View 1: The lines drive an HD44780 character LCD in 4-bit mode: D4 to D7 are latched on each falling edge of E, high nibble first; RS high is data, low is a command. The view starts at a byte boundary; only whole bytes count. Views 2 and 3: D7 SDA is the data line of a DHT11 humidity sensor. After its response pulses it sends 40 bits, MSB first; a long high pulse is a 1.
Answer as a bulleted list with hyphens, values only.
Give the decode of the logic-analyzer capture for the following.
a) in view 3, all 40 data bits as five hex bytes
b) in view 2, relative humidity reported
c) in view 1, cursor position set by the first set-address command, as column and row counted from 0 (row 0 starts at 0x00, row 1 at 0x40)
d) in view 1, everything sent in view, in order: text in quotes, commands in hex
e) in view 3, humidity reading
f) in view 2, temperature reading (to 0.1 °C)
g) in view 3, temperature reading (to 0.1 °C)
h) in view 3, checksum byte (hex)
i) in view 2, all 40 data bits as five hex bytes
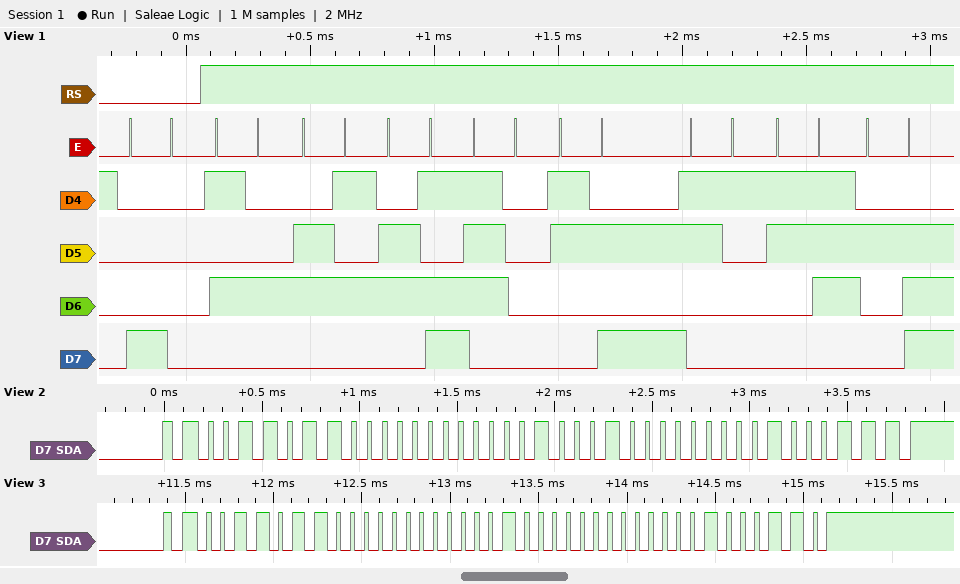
- 36 00 10 00 46
- 54 %
- column 0, row 0
- 0x80 "Temp:17."
- 54 %
- 17.0 °C
- 16.0 °C
- 0x46
- 36 00 11 00 47
